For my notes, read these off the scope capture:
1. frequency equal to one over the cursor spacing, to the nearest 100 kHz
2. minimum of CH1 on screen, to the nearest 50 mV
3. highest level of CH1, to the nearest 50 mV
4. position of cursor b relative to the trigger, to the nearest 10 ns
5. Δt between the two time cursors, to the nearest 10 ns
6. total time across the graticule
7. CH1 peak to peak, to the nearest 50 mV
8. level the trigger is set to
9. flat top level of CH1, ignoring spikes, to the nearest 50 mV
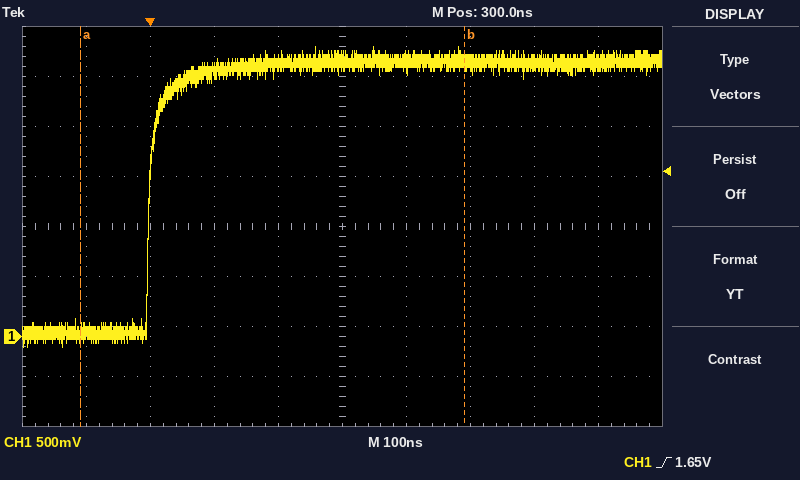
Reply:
1.7 MHz
-100 mV
2.90 V
+490 ns
600 ns
1 µs
3.00 V
1.65 V
2.75 V
